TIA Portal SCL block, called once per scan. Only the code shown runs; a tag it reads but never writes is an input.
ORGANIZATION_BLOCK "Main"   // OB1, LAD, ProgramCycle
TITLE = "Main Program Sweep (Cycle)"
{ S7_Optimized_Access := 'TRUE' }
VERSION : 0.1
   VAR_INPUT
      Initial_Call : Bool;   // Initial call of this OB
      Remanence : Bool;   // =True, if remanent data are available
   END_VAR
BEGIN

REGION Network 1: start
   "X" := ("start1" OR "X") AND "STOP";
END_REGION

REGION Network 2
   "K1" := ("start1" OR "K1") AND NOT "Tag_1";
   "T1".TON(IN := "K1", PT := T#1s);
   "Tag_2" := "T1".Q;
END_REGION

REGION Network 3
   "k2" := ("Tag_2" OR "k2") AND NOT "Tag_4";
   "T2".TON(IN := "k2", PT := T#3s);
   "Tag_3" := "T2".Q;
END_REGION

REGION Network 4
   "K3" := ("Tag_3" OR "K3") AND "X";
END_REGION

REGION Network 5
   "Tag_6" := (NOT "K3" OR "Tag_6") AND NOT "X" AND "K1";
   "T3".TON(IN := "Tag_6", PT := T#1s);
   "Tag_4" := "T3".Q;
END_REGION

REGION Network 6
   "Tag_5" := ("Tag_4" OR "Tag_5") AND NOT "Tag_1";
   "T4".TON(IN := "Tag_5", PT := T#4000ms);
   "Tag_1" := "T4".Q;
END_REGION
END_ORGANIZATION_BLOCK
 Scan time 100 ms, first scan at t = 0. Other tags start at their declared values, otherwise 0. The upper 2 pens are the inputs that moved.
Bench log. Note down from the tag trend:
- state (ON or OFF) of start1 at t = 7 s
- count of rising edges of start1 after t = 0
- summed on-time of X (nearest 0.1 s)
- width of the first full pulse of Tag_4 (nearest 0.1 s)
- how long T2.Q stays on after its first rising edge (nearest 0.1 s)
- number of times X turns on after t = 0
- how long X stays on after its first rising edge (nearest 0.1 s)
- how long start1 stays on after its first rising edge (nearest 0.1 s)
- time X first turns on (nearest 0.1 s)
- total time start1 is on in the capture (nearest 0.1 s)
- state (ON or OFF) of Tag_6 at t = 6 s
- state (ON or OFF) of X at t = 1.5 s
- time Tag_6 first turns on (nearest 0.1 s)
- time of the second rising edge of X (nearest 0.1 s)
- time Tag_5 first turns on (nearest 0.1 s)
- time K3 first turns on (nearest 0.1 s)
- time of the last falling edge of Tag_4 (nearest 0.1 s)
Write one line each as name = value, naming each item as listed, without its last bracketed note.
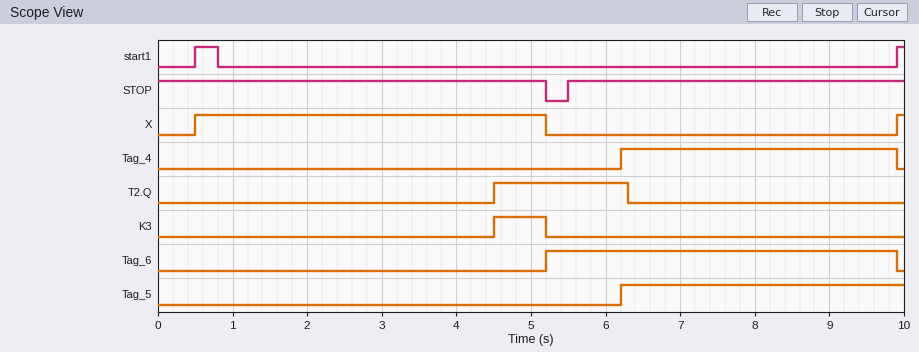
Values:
state (ON or OFF) of start1 at t = 7 s = OFF
count of rising edges of start1 after t = 0 = 2
summed on-time of X = 4.8 s
width of the first full pulse of Tag_4 = 3.7 s
how long T2.Q stays on after its first rising edge = 1.8 s
number of times X turns on after t = 0 = 2
how long X stays on after its first rising edge = 4.7 s
how long start1 stays on after its first rising edge = 0.3 s
time X first turns on = 0.5 s
total time start1 is on in the capture = 0.4 s
state (ON or OFF) of Tag_6 at t = 6 s = ON
state (ON or OFF) of X at t = 1.5 s = ON
time Tag_6 first turns on = 5.2 s
time of the second rising edge of X = 9.9 s
time Tag_5 first turns on = 6.2 s
time K3 first turns on = 4.5 s
time of the last falling edge of Tag_4 = 9.9 s
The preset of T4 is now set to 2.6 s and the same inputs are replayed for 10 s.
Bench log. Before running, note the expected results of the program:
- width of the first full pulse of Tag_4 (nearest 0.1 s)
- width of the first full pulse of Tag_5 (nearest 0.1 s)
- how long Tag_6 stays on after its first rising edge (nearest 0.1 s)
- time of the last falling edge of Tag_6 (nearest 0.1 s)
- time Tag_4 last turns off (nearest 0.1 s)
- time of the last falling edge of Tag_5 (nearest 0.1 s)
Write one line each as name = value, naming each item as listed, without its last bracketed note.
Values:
width of the first full pulse of Tag_4 = 2.7 s
width of the first full pulse of Tag_5 = 2.7 s
how long Tag_6 stays on after its first rising edge = 3.7 s
time of the last falling edge of Tag_6 = 8.9 s
time Tag_4 last turns off = 8.9 s
time of the last falling edge of Tag_5 = 8.9 s
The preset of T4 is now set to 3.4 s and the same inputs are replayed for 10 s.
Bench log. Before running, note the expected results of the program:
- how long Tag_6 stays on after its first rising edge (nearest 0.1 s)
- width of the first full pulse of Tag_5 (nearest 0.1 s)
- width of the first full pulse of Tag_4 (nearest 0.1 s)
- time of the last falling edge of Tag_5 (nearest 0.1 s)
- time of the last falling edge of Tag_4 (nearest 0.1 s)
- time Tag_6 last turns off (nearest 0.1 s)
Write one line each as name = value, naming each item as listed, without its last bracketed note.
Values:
how long Tag_6 stays on after its first rising edge = 4.5 s
width of the first full pulse of Tag_5 = 3.5 s
width of the first full pulse of Tag_4 = 3.5 s
time of the last falling edge of Tag_5 = 9.7 s
time of the last falling edge of Tag_4 = 9.7 s
time Tag_6 last turns off = 9.7 s
